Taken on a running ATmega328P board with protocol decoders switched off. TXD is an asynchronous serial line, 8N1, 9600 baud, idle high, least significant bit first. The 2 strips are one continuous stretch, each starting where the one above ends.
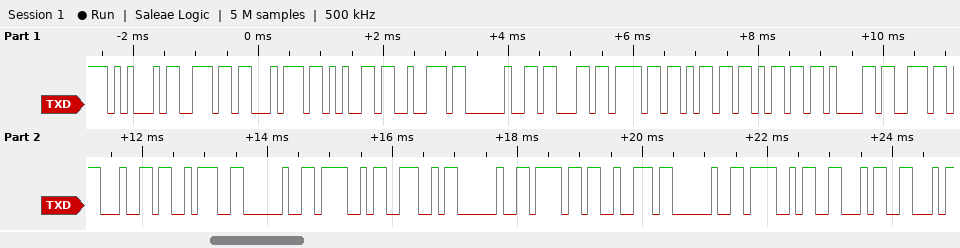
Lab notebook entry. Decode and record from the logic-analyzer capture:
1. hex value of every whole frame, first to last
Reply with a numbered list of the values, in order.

1. 45 6E 74 65 72 20 63 6F 6D 6D 61 6E 64 3A 20 4F 4E 20 6F 72 20 4F 46 46
